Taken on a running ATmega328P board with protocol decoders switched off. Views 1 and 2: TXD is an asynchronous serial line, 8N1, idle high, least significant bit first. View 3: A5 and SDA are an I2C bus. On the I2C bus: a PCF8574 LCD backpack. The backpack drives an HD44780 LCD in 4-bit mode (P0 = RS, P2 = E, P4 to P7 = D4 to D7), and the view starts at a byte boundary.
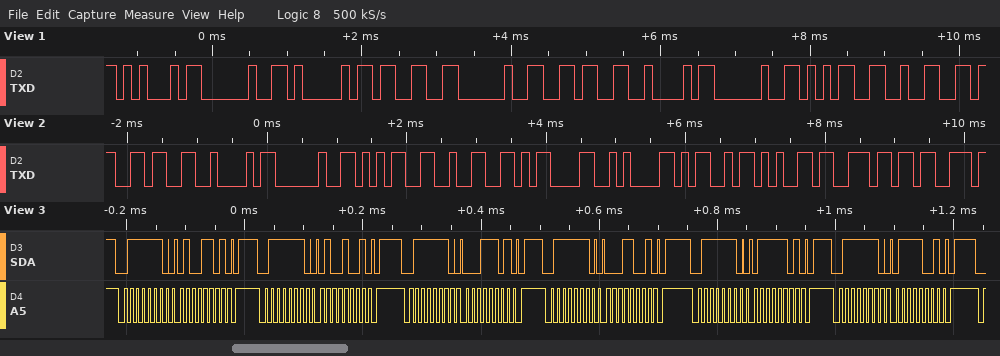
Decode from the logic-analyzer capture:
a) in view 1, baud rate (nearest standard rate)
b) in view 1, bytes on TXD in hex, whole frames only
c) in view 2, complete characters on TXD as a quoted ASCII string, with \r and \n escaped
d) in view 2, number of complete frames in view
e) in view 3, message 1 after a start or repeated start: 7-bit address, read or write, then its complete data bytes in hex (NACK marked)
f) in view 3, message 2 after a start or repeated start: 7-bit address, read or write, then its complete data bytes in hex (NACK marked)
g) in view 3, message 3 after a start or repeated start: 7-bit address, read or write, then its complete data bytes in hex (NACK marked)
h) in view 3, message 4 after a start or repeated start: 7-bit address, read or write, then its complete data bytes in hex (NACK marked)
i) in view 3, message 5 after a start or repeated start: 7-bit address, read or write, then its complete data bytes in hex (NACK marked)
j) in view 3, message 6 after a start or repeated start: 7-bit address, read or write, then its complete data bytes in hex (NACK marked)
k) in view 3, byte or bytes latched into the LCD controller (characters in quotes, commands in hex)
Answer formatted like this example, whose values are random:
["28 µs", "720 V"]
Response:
["9600 baud", "45 20 41 33 20 36 42 20 35 32", "\"6B 52\\r\\nMens\"", "11", "0x3F write: 4D", "0x3F write: 49", "0x3F write: 1D", "0x3F write: 19", "0x3F write: 7D", "0x3F write: 79", "'A'"]
